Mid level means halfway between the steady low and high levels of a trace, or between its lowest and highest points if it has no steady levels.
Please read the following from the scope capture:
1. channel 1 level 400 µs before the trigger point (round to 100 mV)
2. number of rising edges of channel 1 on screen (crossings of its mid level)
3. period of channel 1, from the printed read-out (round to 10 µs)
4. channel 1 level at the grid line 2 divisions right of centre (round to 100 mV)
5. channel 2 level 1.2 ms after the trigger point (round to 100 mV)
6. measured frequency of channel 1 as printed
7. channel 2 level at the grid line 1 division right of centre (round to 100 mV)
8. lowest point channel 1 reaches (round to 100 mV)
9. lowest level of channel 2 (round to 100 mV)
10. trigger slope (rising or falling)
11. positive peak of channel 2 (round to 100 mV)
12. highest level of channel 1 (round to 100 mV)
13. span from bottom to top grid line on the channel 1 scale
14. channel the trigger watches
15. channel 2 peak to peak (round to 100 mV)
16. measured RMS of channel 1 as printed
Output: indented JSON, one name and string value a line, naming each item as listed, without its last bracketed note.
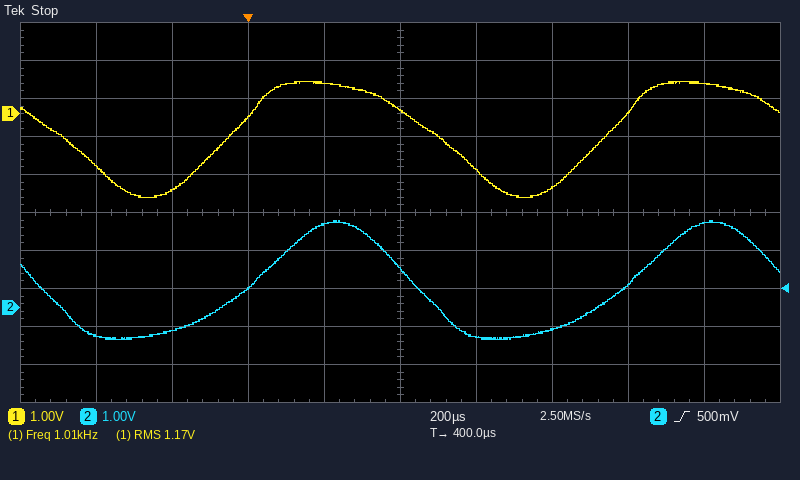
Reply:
{
  "channel 1 level 400 µs before the trigger point": "-1.4 V",
  "number of rising edges of channel 1 on screen": "2",
  "period of channel 1, from the printed read-out": "990 µs",
  "channel 1 level at the grid line 2 divisions right of centre": "-1.9 V",
  "channel 2 level 1.2 ms after the trigger point": "2.2 V",
  "measured frequency of channel 1 as printed": "1.01 kHz",
  "channel 2 level at the grid line 1 division right of centre": "-800 mV",
  "lowest point channel 1 reaches": "-2.2 V",
  "lowest level of channel 2": "-800 mV",
  "trigger slope": "rising",
  "positive peak of channel 2": "2.3 V",
  "highest level of channel 1": "800 mV",
  "span from bottom to top grid line on the channel 1 scale": "10 V",
  "channel the trigger watches": "channel 2",
  "channel 2 peak to peak": "3.1 V",
  "measured RMS of channel 1 as printed": "1.17 V"
}
